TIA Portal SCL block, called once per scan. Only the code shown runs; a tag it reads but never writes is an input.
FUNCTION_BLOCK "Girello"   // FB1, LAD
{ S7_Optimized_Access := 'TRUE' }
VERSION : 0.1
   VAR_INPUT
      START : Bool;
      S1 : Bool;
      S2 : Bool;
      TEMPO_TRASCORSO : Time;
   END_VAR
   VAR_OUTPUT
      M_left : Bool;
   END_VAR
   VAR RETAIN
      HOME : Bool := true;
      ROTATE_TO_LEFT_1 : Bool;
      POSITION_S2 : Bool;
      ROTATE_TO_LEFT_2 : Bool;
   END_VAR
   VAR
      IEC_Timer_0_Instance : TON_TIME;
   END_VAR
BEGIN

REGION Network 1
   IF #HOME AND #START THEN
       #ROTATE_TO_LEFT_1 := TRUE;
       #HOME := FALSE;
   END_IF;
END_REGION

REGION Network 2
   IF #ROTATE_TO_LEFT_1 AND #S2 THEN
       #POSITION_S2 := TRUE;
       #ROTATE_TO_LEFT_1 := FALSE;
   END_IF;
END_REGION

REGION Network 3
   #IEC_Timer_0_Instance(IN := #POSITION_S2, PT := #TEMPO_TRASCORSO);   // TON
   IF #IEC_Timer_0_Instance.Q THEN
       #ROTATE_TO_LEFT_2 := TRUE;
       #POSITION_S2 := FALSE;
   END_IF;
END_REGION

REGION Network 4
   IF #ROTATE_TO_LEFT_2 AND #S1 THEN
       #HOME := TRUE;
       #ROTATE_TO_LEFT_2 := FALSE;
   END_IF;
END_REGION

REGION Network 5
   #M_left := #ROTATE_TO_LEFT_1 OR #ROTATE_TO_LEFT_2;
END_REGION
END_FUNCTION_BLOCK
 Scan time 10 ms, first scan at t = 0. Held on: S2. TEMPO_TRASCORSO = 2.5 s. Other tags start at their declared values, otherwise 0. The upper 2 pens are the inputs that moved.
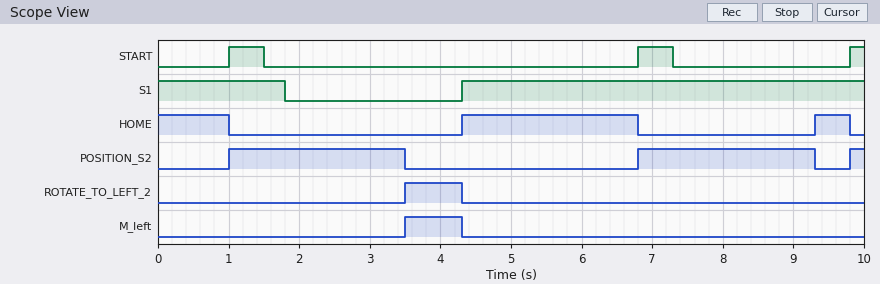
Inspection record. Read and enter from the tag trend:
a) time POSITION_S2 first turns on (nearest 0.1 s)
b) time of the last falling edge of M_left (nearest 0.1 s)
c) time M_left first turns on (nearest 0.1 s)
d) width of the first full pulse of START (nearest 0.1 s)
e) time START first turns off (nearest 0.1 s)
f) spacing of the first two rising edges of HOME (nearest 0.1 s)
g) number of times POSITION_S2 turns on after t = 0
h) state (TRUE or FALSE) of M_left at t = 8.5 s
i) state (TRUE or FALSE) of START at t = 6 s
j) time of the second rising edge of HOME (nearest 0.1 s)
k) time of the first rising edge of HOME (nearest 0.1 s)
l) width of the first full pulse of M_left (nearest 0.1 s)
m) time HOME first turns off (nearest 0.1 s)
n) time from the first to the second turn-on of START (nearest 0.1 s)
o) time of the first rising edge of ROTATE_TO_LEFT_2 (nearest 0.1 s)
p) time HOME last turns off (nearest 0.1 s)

1.0 s
4.3 s
3.5 s
0.5 s
1.5 s
5.0 s
3
FALSE
FALSE
9.3 s
4.3 s
0.8 s
1.0 s
5.8 s
3.5 s
9.8 s
